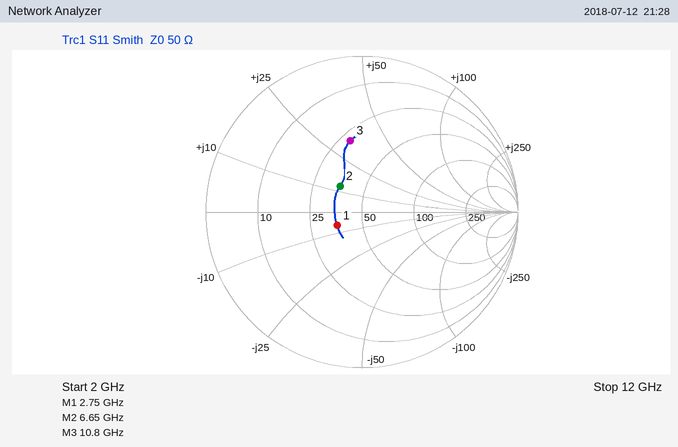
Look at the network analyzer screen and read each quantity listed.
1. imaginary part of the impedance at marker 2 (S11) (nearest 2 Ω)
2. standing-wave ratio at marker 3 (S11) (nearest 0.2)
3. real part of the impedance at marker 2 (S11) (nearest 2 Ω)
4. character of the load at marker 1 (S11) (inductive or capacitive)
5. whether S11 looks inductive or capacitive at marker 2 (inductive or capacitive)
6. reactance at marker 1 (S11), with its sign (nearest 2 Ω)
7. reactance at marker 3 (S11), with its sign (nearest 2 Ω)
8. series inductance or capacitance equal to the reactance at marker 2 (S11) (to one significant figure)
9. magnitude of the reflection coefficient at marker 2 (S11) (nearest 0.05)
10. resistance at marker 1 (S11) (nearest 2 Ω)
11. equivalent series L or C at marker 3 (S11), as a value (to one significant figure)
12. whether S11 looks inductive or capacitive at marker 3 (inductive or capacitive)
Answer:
+12 Ω
2.8
36 Ω
capacitive
inductive
-6 Ω
+34 Ω
300 pH
0.20
36 Ω
500 pH
inductive
